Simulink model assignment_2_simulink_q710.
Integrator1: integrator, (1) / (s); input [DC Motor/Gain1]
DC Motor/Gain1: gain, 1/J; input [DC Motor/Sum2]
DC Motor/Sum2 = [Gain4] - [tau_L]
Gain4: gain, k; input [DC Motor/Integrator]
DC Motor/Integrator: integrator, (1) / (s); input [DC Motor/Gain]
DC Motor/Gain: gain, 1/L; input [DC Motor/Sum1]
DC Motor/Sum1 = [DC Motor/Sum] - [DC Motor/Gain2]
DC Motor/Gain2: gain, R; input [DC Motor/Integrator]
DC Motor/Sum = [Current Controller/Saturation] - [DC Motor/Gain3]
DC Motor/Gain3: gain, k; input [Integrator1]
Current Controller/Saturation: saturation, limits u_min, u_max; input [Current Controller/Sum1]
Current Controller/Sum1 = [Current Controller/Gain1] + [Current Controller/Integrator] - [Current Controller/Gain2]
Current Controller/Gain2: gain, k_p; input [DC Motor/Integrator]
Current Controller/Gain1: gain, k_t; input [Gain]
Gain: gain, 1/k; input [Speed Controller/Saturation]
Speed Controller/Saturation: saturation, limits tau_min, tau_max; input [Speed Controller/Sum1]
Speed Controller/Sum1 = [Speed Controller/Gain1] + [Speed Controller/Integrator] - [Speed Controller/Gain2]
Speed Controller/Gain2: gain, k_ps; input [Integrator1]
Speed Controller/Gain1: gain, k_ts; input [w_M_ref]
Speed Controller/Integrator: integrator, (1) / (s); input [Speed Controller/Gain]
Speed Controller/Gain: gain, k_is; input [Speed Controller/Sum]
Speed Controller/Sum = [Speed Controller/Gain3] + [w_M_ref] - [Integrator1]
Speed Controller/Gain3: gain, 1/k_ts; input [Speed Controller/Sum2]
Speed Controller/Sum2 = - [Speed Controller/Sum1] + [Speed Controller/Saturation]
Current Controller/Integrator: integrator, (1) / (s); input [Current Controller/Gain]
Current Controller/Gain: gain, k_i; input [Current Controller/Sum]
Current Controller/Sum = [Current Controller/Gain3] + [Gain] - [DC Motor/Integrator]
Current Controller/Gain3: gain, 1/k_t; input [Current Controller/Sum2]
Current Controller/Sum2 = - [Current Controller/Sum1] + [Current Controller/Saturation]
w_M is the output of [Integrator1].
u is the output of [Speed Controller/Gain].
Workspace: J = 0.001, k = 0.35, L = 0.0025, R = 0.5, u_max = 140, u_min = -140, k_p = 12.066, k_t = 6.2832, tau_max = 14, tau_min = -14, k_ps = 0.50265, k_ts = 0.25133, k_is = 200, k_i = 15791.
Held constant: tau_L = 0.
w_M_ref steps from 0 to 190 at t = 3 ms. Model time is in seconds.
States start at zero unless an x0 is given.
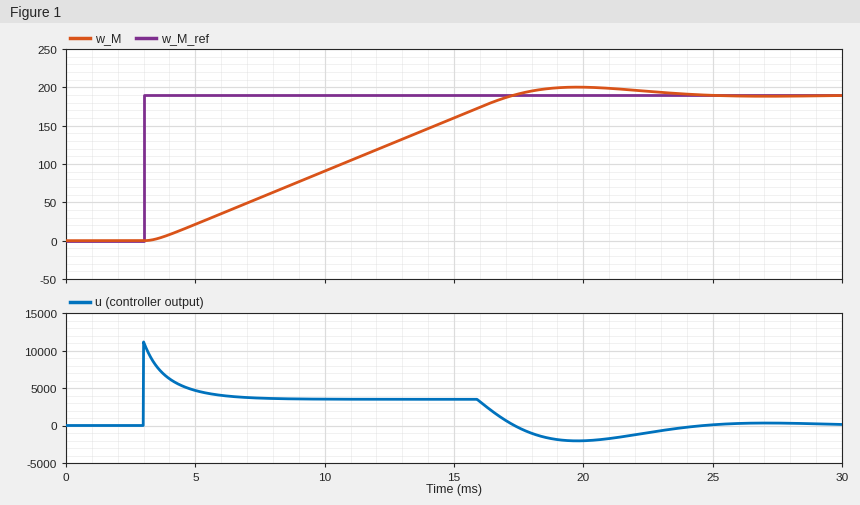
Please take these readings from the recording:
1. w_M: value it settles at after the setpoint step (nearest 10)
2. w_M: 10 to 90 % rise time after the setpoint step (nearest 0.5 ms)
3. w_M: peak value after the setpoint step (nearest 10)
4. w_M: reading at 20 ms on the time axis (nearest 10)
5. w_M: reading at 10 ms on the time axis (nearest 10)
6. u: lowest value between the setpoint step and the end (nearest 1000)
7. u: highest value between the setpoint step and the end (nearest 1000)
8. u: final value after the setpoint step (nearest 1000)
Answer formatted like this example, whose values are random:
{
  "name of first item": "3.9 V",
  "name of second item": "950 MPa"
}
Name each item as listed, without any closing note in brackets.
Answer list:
{
  "w_M: value it settles at after the setpoint step": "190",
  "w_M: 10 to 90 % rise time after the setpoint step": "11.0 ms",
  "w_M: peak value after the setpoint step": "200",
  "w_M: reading at 20 ms on the time axis": "200",
  "w_M: reading at 10 ms on the time axis": "90",
  "u: lowest value between the setpoint step and the end": "-2000",
  "u: highest value between the setpoint step and the end": "11000",
  "u: final value after the setpoint step": "0"
}
